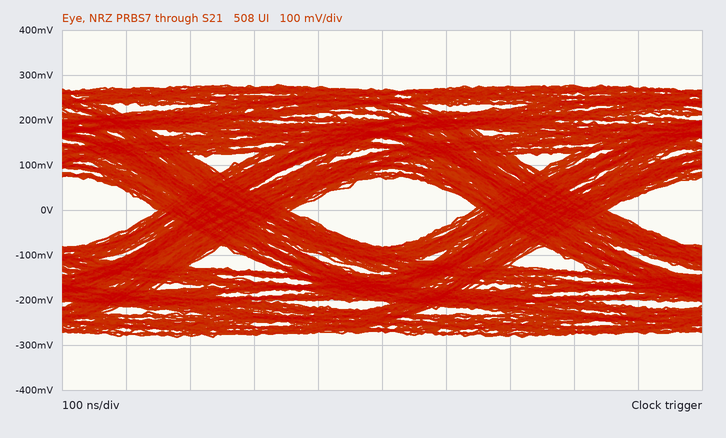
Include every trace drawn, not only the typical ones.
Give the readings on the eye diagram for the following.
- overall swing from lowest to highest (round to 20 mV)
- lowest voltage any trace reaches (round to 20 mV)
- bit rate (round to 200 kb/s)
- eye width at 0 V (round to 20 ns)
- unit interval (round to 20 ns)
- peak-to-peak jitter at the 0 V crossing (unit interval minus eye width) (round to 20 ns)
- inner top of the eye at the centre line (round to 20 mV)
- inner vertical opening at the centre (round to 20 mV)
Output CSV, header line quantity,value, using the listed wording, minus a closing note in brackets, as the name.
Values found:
quantity,value
overall swing from lowest to highest,560 mV
lowest voltage any trace reaches,-280 mV
bit rate,2.0 Mb/s
eye width at 0 V,280 ns
unit interval,500 ns
peak-to-peak jitter at the 0 V crossing (unit interval minus eye width),220 ns
inner top of the eye at the centre line,80 mV
inner vertical opening at the centre,160 mV
